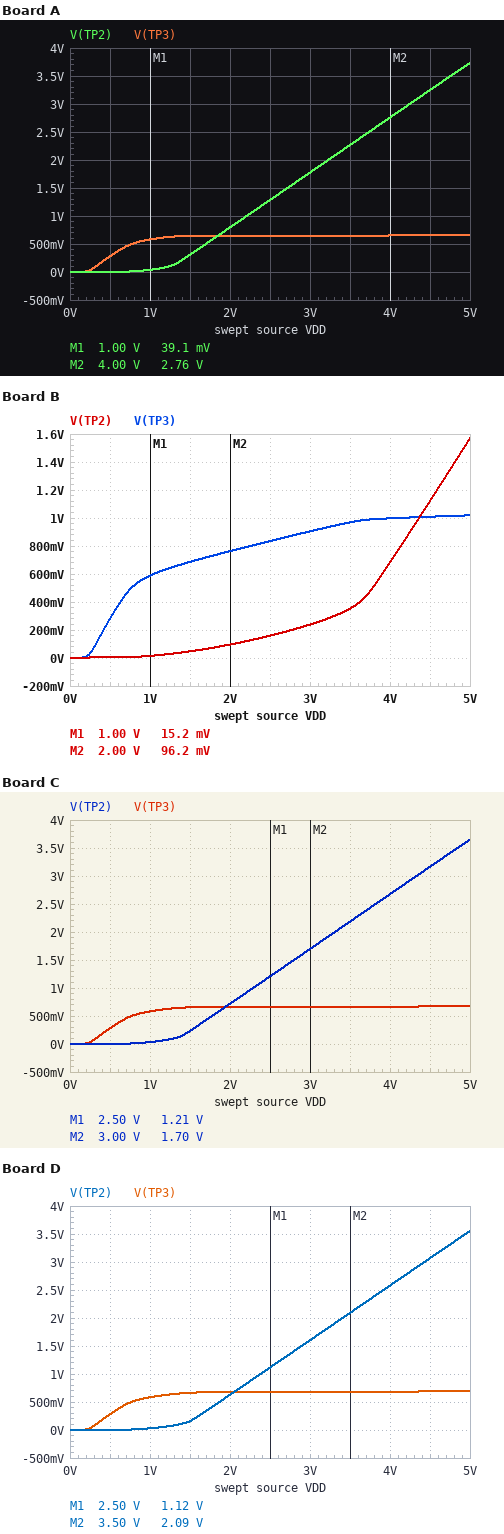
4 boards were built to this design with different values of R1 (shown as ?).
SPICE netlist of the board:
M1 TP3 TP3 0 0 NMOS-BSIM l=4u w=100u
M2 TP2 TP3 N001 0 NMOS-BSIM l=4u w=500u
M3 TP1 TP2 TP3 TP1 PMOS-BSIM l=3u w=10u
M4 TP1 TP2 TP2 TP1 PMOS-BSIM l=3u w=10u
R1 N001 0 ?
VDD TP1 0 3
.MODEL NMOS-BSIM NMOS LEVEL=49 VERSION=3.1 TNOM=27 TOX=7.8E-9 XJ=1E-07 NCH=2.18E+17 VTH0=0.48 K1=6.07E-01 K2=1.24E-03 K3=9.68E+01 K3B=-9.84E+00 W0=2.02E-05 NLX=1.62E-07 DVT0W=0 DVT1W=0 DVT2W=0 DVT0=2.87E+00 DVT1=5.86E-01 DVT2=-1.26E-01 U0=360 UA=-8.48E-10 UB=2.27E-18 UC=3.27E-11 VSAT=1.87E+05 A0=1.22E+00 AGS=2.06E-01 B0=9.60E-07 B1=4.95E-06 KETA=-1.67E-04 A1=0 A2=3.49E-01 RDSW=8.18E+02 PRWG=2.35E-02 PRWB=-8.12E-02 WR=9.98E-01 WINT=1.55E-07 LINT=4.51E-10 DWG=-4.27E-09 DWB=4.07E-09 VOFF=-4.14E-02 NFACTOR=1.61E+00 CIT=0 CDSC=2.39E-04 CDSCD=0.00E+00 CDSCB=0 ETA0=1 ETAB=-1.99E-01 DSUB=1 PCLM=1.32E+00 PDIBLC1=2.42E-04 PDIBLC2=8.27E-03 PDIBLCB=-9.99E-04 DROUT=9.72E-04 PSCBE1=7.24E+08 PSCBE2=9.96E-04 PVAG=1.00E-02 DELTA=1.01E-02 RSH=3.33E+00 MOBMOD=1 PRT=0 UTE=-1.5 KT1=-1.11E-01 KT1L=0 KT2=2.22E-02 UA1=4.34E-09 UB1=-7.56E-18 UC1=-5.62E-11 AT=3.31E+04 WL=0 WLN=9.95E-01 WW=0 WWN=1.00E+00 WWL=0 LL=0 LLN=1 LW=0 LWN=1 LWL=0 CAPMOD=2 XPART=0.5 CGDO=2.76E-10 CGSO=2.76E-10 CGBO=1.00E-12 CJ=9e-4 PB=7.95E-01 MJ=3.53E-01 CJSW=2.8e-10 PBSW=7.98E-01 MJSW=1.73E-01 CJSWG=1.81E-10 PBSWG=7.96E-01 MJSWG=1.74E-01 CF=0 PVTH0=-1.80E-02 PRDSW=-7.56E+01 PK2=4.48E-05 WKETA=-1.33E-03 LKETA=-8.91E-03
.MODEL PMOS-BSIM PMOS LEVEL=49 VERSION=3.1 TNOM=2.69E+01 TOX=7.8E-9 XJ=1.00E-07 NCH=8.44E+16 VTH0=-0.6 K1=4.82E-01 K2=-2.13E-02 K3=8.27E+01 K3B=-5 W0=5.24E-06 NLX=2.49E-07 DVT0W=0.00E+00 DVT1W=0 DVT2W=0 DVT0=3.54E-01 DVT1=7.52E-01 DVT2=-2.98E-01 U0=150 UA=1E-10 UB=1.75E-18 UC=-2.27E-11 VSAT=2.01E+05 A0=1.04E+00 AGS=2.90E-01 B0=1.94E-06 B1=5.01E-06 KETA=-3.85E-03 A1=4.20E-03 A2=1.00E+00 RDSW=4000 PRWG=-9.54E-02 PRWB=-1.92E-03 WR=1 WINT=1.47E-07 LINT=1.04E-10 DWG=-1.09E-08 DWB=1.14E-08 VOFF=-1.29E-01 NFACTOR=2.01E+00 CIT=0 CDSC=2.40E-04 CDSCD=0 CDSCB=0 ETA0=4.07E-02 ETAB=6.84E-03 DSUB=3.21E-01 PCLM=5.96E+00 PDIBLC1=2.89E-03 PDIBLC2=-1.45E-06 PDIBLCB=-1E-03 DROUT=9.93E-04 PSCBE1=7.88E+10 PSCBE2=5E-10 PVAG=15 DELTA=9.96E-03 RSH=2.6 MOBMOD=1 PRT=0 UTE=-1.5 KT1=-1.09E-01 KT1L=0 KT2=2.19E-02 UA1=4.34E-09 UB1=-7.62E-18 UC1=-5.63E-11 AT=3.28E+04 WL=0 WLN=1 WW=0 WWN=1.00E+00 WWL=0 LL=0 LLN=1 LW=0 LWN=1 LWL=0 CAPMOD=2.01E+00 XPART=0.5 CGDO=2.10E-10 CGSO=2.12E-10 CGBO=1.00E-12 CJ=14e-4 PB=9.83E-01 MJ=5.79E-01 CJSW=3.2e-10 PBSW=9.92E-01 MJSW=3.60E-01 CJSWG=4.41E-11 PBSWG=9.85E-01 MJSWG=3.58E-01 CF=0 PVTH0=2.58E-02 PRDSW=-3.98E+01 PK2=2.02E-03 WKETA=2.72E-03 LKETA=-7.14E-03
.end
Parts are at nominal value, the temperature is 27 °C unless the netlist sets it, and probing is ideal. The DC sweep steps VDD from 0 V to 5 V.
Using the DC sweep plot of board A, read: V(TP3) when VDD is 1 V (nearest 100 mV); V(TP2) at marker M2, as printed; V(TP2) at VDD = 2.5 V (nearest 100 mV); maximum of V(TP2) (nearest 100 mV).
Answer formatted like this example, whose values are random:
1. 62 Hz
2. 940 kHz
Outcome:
1. 600 mV
2. 2.76 V
3. 1.3 V
4. 3.7 V
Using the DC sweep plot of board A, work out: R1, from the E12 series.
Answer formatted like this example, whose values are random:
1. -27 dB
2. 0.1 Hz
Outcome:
1. 2.7 kΩ
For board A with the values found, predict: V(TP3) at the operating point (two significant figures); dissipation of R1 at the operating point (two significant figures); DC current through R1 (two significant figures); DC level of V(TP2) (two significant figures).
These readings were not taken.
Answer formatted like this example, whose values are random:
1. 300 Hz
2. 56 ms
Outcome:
1. 650 mV
2. 2.0 µW
3. 27 µA
4. 1.8 V
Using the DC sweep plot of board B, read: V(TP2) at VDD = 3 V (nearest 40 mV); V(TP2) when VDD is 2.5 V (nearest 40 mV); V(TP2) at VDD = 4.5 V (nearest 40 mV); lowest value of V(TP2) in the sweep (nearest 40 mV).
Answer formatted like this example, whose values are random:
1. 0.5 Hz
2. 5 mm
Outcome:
1. 240 mV
2. 160 mV
3. 1.12 V
4. 0 V
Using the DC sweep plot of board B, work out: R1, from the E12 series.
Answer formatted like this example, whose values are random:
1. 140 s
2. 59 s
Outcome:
1. 470 Ω
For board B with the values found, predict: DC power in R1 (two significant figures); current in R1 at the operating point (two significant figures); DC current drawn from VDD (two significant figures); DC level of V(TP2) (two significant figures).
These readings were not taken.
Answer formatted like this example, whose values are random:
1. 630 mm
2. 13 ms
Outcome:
1. 41 µW
2. 290 µA
3. 580 µA
4. 240 mV
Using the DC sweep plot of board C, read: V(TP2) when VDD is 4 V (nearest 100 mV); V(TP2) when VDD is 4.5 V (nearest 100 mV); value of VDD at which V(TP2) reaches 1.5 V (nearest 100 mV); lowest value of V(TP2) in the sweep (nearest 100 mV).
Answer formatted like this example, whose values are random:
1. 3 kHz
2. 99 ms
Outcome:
1. 2.7 V
2. 3.2 V
3. 2.8 V
4. 0 V
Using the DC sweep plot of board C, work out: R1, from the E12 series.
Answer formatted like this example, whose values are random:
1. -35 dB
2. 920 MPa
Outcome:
1. 2.2 kΩ
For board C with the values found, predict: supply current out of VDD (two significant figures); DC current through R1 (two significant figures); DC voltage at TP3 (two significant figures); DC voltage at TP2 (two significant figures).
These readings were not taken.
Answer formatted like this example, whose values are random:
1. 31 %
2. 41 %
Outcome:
1. 70 µA
2. 35 µA
3. 660 mV
4. 1.7 V
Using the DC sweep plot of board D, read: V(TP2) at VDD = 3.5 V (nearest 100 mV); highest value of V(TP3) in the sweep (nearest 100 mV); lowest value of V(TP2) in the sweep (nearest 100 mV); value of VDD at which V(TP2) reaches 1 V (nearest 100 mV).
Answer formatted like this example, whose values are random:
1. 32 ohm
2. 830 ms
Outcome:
1. 2.1 V
2. 700 mV
3. 0 V
4. 2.4 V
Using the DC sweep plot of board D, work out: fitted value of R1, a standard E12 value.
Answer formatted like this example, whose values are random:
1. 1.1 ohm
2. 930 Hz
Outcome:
1. 1.8 kΩ
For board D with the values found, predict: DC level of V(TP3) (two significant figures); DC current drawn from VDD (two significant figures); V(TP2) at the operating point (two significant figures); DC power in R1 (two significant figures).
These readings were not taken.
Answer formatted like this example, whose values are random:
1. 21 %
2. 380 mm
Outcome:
1. 680 mV
2. 90 µA
3. 1.6 V
4. 3.6 µW
